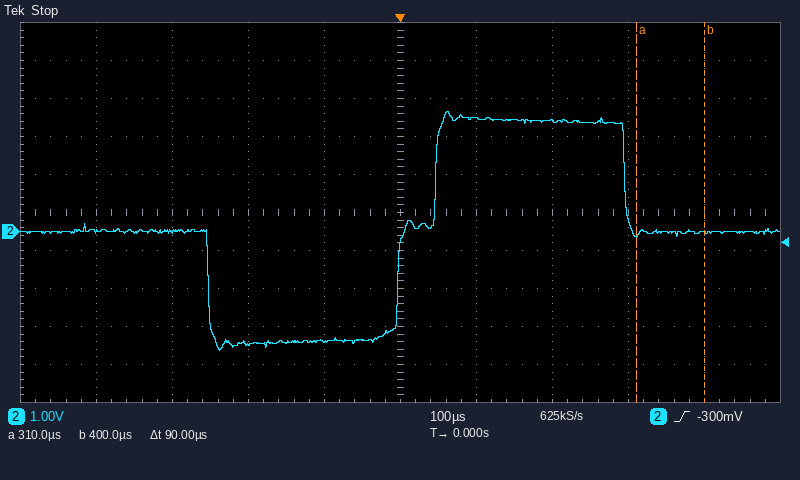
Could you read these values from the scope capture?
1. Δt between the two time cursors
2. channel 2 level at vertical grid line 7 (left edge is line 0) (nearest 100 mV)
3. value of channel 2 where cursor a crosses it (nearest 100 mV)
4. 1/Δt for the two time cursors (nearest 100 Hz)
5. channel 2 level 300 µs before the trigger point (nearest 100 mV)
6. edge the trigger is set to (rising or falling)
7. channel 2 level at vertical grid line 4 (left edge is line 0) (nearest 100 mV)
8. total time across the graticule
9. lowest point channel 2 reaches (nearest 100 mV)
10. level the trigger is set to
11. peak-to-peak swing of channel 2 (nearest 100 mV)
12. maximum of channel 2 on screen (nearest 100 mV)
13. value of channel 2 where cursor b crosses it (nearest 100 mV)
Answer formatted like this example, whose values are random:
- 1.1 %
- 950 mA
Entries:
- 90 µs
- 2.9 V
- -100 mV
- 11.1 kHz
- 0.0 V
- rising
- -2.9 V
- 1 ms
- -3.1 V
- -300 mV
- 6.3 V
- 3.2 V
- 0.0 V
